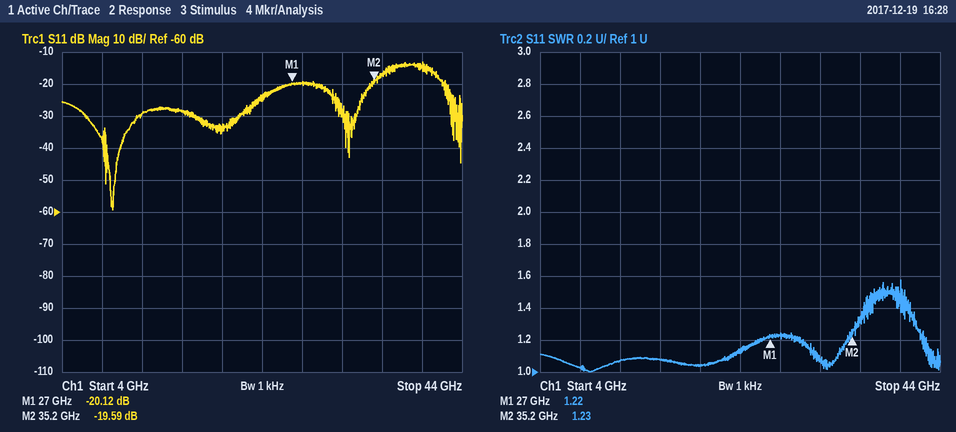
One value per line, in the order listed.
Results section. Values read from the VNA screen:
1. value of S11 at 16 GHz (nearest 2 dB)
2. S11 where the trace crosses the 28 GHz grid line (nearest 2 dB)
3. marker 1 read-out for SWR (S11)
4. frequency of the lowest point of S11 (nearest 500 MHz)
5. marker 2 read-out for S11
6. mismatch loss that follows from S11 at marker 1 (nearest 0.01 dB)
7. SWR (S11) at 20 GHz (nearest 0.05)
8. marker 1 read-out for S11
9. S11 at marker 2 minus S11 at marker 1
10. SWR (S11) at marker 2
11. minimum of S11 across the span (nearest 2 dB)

-28 dB
-20 dB
1.22
9.0 GHz
-19.59 dB
0.04 dB
1.05
-20.12 dB
0.53 dB
1.23
-60 dB
